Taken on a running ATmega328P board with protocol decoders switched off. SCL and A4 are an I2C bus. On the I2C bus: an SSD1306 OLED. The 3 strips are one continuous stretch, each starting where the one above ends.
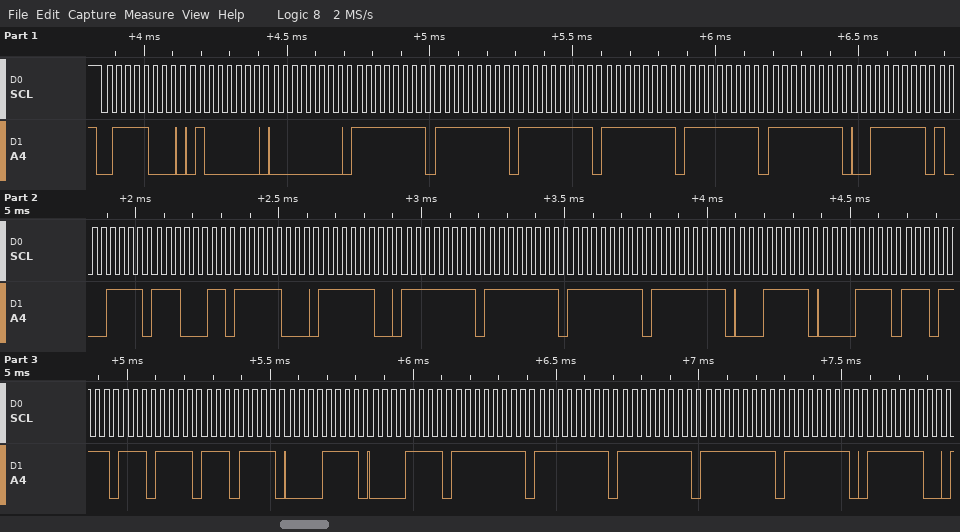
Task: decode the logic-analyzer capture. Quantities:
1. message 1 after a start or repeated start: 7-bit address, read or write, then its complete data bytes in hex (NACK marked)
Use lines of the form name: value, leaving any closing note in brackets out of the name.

message 1 after a start or repeated start: 7-bit address, read or write, then its complete data bytes in hex: 0x3C write: 40 00 FF FF FF FF FF FF 3F 8F E3 F8 FC FF FF FF FF 1F 0F EF EF EF 0F 0F FF FF FF FF FE FC
